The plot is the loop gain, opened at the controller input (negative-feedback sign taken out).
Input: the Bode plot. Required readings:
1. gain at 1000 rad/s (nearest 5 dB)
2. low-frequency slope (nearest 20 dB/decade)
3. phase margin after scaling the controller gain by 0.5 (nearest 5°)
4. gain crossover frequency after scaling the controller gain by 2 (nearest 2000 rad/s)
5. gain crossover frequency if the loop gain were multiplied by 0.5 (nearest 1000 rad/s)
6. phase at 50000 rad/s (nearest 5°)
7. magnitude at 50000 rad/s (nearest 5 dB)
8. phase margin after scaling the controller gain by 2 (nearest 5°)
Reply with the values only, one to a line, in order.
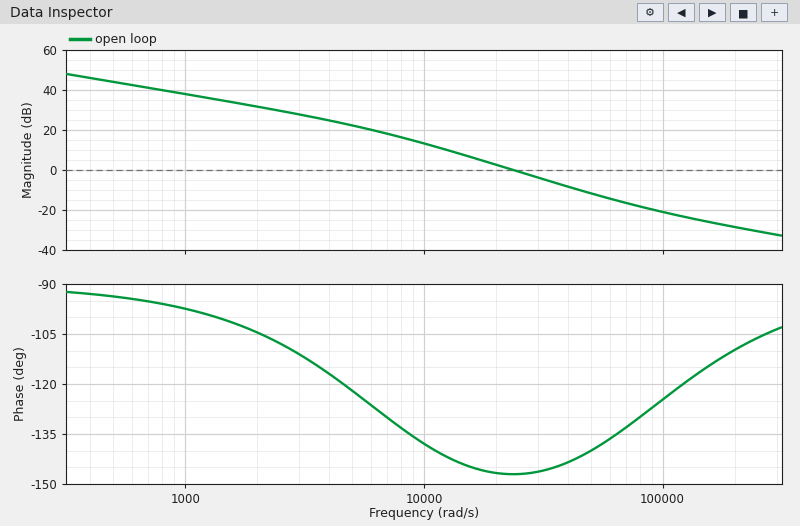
40 dB
-20 dB/decade
35°
34000 rad/s
16000 rad/s
-140°
-10 dB
35°
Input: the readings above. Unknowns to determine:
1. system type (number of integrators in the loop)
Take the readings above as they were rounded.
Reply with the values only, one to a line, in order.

1
